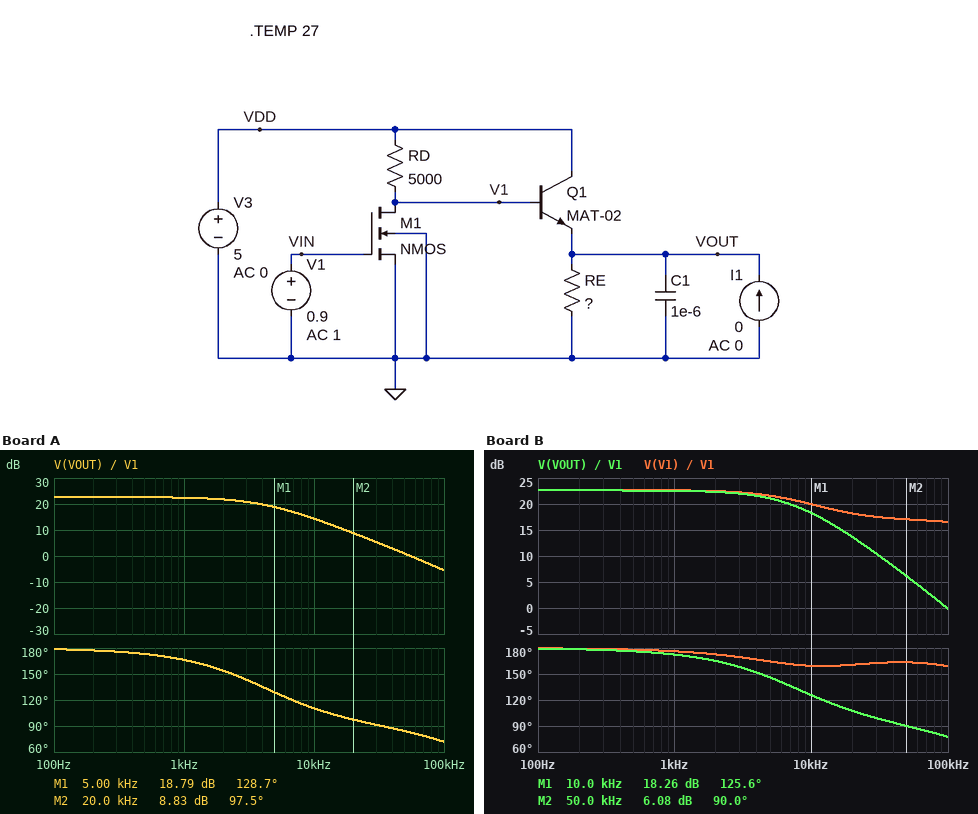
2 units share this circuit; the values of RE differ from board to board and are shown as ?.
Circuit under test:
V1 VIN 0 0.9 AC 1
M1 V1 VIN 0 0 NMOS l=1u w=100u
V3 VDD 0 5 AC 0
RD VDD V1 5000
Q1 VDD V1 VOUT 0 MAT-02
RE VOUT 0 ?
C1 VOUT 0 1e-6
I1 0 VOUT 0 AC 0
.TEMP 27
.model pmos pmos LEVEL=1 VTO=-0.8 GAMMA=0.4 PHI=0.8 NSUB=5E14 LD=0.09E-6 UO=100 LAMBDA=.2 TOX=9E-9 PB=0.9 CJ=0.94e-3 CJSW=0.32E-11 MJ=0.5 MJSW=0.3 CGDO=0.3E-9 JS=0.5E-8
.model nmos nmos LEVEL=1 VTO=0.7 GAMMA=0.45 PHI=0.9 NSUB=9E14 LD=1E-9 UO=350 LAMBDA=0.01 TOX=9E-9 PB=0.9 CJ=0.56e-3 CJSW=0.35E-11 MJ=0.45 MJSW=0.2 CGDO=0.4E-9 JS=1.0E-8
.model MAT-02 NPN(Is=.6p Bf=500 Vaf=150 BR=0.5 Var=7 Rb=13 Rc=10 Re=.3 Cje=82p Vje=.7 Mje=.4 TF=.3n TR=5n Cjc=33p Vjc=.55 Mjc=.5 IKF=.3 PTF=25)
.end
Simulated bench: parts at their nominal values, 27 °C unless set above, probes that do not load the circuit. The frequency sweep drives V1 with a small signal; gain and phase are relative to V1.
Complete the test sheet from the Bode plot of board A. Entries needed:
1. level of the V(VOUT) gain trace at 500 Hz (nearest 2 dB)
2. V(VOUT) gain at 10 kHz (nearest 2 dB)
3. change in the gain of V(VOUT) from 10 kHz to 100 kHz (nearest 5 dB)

22 dB
14 dB
-20 dB
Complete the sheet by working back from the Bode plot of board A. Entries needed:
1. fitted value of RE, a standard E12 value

3.3 kΩ
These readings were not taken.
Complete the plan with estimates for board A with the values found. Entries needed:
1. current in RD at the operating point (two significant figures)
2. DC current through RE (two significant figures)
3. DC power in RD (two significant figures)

280 µA
920 µA
390 µW
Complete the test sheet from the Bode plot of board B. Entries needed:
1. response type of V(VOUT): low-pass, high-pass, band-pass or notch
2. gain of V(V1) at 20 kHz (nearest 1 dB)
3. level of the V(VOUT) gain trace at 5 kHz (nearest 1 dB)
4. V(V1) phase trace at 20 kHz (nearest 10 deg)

low-pass
18 dB
21 dB
160 deg
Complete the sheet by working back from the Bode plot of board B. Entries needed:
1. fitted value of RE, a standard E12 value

1.2 kΩ
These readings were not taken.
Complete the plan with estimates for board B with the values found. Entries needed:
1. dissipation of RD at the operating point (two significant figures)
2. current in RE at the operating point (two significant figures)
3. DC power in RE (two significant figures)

400 µW
2.5 mA
7.5 mW
